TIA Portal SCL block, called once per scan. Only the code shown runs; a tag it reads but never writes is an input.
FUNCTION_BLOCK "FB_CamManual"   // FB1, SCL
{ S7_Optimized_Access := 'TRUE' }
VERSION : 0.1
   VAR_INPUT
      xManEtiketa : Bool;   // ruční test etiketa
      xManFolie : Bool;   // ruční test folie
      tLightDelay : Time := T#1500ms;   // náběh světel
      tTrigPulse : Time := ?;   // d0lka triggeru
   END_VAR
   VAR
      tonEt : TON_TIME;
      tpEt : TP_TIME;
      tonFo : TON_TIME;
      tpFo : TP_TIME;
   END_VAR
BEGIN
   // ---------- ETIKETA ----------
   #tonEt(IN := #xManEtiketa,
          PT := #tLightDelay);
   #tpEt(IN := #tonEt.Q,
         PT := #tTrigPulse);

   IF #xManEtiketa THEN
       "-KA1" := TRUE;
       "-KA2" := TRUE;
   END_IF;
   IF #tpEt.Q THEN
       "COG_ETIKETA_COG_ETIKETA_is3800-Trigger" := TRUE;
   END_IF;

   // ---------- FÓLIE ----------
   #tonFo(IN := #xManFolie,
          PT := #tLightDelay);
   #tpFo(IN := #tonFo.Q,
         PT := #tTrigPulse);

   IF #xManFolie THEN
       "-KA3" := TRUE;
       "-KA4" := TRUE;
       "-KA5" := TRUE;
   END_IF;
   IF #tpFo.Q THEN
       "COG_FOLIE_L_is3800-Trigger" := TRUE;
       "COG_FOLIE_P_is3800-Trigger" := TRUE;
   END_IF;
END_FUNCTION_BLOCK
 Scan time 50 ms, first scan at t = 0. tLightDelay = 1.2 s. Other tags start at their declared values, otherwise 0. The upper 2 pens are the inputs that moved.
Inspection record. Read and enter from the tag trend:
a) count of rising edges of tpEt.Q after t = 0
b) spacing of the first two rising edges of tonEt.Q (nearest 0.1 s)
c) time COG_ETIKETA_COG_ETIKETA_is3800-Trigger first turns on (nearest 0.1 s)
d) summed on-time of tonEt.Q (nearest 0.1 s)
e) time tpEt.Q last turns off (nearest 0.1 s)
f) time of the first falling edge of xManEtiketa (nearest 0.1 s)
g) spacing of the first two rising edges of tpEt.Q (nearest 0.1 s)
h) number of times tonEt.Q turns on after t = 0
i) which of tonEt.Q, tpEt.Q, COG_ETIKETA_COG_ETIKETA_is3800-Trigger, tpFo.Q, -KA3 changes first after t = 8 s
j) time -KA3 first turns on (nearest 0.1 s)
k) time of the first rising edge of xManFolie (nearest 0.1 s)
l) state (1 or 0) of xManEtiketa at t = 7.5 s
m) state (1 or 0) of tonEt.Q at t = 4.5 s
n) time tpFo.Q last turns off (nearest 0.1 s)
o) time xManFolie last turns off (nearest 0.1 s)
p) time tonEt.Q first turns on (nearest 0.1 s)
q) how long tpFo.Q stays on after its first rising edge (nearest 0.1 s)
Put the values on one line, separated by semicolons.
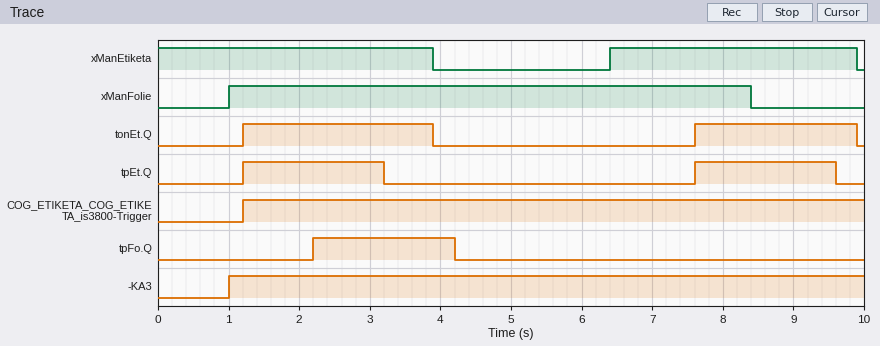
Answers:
2; 6.4 s; 1.2 s; 5.0 s; 9.6 s; 3.9 s; 6.4 s; 2; tpEt.Q; 1.0 s; 1.0 s; 1; 0; 4.2 s; 8.4 s; 1.2 s; 2.0 s
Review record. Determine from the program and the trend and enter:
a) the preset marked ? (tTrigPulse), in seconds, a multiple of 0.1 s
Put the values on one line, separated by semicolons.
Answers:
2.0 s
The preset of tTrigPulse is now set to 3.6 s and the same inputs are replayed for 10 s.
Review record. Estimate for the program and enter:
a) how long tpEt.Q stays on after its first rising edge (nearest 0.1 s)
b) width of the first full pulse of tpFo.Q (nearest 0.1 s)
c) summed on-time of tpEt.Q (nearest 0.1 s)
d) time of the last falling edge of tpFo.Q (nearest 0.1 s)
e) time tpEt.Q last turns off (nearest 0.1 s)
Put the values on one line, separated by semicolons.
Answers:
3.6 s; 3.6 s; 6.0 s; 5.8 s; 4.8 s
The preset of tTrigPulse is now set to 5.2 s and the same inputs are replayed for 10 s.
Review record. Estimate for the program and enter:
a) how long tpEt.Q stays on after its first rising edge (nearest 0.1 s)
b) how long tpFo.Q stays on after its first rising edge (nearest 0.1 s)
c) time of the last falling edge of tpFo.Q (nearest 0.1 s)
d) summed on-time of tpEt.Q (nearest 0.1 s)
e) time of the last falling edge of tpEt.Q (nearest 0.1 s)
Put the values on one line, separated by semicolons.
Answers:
5.2 s; 5.2 s; 7.4 s; 7.6 s; 6.4 s
